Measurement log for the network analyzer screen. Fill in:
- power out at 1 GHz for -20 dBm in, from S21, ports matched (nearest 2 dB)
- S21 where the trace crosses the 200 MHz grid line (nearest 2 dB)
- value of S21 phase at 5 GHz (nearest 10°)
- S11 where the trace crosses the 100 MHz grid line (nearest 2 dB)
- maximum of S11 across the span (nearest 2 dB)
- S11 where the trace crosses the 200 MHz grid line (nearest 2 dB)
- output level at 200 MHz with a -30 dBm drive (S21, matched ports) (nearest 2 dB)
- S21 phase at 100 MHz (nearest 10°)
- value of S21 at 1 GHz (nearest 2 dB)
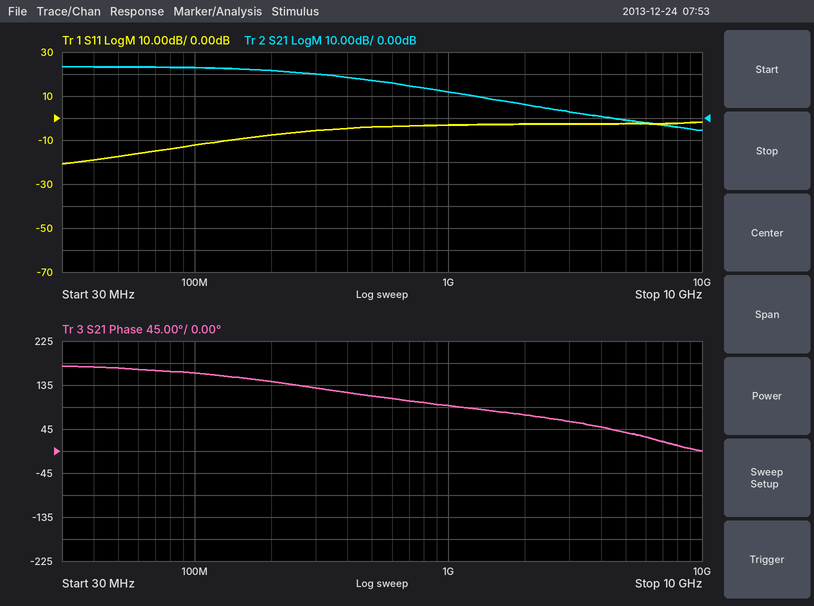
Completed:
-8 dBm
22 dB
40°
-12 dB
-2 dB
-8 dB
-8 dBm
160°
12 dB
